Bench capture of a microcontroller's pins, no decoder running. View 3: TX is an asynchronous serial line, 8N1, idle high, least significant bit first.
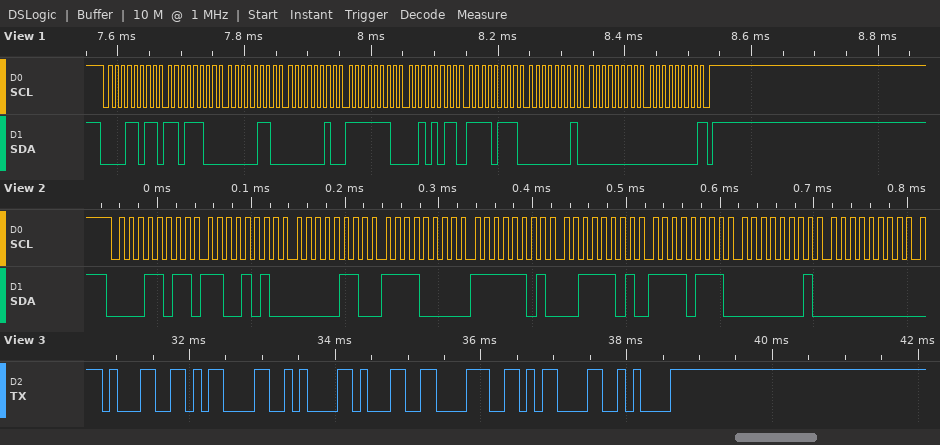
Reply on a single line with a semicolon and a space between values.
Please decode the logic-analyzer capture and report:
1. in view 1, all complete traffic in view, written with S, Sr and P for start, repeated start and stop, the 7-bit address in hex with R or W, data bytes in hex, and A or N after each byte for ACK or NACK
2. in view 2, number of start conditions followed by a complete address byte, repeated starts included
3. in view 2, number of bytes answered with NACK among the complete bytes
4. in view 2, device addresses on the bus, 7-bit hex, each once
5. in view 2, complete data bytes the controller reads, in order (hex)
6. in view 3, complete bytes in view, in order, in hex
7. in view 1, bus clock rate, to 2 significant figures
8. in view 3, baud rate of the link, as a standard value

S 0DR A DC A 06 A 02 A FE A 2B A F7 A 01 A 00 A 00 N P; 1; 0; 0x0D; CA 06 F0 FD 3D F7 01 00; 31 0D 0A 31 38 0D 0A; 100 kHz; 9600 baud
